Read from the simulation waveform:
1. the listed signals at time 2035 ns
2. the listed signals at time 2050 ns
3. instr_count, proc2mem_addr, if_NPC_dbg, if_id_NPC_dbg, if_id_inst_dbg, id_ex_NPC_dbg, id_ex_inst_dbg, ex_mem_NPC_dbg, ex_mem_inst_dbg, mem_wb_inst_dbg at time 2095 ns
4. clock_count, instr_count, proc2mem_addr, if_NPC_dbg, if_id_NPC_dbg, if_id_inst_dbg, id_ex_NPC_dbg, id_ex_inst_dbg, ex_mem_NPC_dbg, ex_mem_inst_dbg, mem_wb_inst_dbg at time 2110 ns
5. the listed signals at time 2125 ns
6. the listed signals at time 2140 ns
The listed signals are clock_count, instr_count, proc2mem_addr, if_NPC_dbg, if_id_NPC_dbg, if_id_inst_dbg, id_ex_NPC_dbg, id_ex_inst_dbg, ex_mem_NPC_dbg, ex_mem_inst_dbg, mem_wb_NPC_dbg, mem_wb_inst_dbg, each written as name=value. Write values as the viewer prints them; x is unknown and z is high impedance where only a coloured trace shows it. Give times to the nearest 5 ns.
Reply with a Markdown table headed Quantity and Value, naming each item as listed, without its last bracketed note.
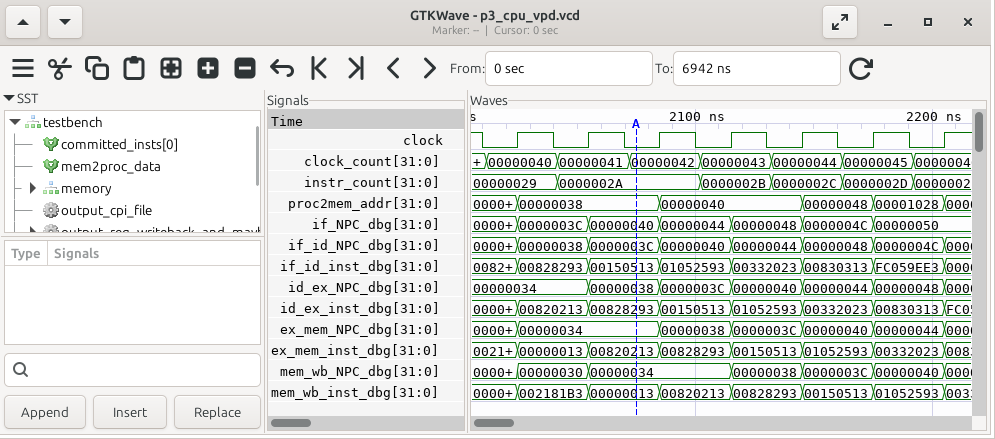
| Quantity | Value |
|---|---|
| the listed signals at time 2035 ns | clock_count=00000040, instr_count=00000029, proc2mem_addr=00000038, if_NPC_dbg=0000003C, if_id_NPC_dbg=00000038, if_id_inst_dbg=00828293, id_ex_NPC_dbg=00000034, id_ex_inst_dbg=00820213, ex_mem_NPC_dbg=00000034, ex_mem_inst_dbg=00000013, mem_wb_NPC_dbg=00000030, mem_wb_inst_dbg=002181B3 |
| the listed signals at time 2050 ns | clock_count=00000041, instr_count=0000002A, proc2mem_addr=00000038, if_NPC_dbg=0000003C, if_id_NPC_dbg=00000038, if_id_inst_dbg=00828293, id_ex_NPC_dbg=00000034, id_ex_inst_dbg=00820213, ex_mem_NPC_dbg=00000034, ex_mem_inst_dbg=00000013, mem_wb_NPC_dbg=00000030, mem_wb_inst_dbg=002181B3 |
| instr_count, proc2mem_addr, if_NPC_dbg, if_id_NPC_dbg, if_id_inst_dbg, id_ex_NPC_dbg, id_ex_inst_dbg, ex_mem_NPC_dbg, ex_mem_inst_dbg, mem_wb_inst_dbg at time 2095 ns | instr_count=0000002A, proc2mem_addr=00000040, if_NPC_dbg=00000044, if_id_NPC_dbg=00000040, if_id_inst_dbg=01052593, id_ex_NPC_dbg=0000003C, id_ex_inst_dbg=00150513, ex_mem_NPC_dbg=00000038, ex_mem_inst_dbg=00828293, mem_wb_inst_dbg=00820213 |
| clock_count, instr_count, proc2mem_addr, if_NPC_dbg, if_id_NPC_dbg, if_id_inst_dbg, id_ex_NPC_dbg, id_ex_inst_dbg, ex_mem_NPC_dbg, ex_mem_inst_dbg, mem_wb_inst_dbg at time 2110 ns | clock_count=00000043, instr_count=0000002B, proc2mem_addr=00000040, if_NPC_dbg=00000044, if_id_NPC_dbg=00000040, if_id_inst_dbg=01052593, id_ex_NPC_dbg=0000003C, id_ex_inst_dbg=00150513, ex_mem_NPC_dbg=00000038, ex_mem_inst_dbg=00828293, mem_wb_inst_dbg=00820213 |
| the listed signals at time 2125 ns | clock_count=00000043, instr_count=0000002B, proc2mem_addr=00000040, if_NPC_dbg=00000048, if_id_NPC_dbg=00000044, if_id_inst_dbg=00332023, id_ex_NPC_dbg=00000040, id_ex_inst_dbg=01052593, ex_mem_NPC_dbg=0000003C, ex_mem_inst_dbg=00150513, mem_wb_NPC_dbg=00000038, mem_wb_inst_dbg=00828293 |
| the listed signals at time 2140 ns | clock_count=00000044, instr_count=0000002C, proc2mem_addr=00000040, if_NPC_dbg=00000048, if_id_NPC_dbg=00000044, if_id_inst_dbg=00332023, id_ex_NPC_dbg=00000040, id_ex_inst_dbg=01052593, ex_mem_NPC_dbg=0000003C, ex_mem_inst_dbg=00150513, mem_wb_NPC_dbg=00000038, mem_wb_inst_dbg=00828293 |
